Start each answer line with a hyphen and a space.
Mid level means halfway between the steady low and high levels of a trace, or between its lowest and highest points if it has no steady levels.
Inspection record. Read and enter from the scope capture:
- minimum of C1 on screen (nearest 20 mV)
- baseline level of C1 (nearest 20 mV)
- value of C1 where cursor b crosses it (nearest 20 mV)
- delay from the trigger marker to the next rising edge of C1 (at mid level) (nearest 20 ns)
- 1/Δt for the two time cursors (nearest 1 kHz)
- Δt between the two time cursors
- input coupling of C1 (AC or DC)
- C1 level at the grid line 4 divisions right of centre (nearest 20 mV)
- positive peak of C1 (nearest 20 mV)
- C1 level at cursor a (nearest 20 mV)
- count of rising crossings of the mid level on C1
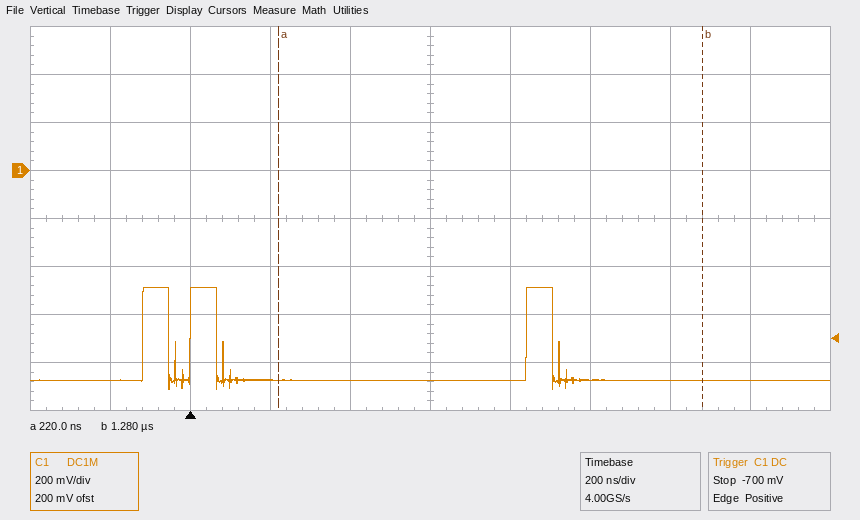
- -920 mV
- -880 mV
- -880 mV
- 840 ns
- 943 kHz
- 1.06 µs
- DC
- -880 mV
- -480 mV
- -880 mV
- 3
